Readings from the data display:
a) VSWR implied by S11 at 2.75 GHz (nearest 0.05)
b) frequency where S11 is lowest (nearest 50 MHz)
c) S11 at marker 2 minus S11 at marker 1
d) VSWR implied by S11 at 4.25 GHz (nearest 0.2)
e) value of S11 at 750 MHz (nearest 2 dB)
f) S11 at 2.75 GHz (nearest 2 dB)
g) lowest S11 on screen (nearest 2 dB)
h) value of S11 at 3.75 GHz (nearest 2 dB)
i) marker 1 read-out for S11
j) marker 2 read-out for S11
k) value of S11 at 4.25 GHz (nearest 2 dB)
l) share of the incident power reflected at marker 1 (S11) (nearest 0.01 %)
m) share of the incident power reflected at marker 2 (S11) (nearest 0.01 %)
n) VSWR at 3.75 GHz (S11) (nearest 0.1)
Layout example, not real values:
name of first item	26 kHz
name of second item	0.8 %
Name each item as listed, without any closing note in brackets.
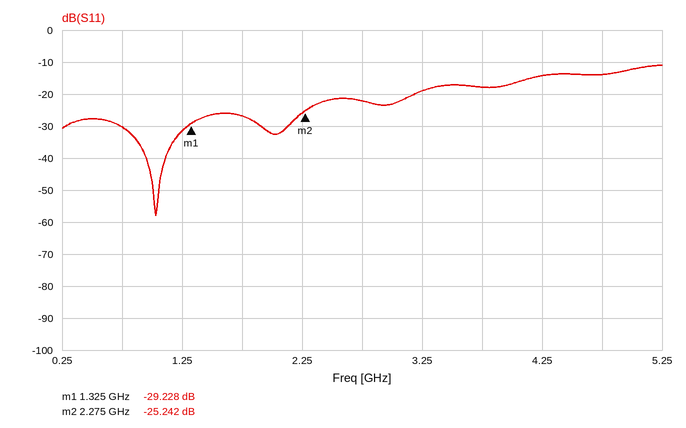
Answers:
VSWR implied by S11 at 2.75 GHz	1.15
frequency where S11 is lowest	1.05 GHz
S11 at marker 2 minus S11 at marker 1	3.986 dB
VSWR implied by S11 at 4.25 GHz	1.4
value of S11 at 750 MHz	-30 dB
S11 at 2.75 GHz	-22 dB
lowest S11 on screen	-58 dB
value of S11 at 3.75 GHz	-18 dB
marker 1 read-out for S11	-29.228 dB
marker 2 read-out for S11	-25.242 dB
value of S11 at 4.25 GHz	-14 dB
share of the incident power reflected at marker 1 (S11)	0.12 %
share of the incident power reflected at marker 2 (S11)	0.30 %
VSWR at 3.75 GHz (S11)	1.3
